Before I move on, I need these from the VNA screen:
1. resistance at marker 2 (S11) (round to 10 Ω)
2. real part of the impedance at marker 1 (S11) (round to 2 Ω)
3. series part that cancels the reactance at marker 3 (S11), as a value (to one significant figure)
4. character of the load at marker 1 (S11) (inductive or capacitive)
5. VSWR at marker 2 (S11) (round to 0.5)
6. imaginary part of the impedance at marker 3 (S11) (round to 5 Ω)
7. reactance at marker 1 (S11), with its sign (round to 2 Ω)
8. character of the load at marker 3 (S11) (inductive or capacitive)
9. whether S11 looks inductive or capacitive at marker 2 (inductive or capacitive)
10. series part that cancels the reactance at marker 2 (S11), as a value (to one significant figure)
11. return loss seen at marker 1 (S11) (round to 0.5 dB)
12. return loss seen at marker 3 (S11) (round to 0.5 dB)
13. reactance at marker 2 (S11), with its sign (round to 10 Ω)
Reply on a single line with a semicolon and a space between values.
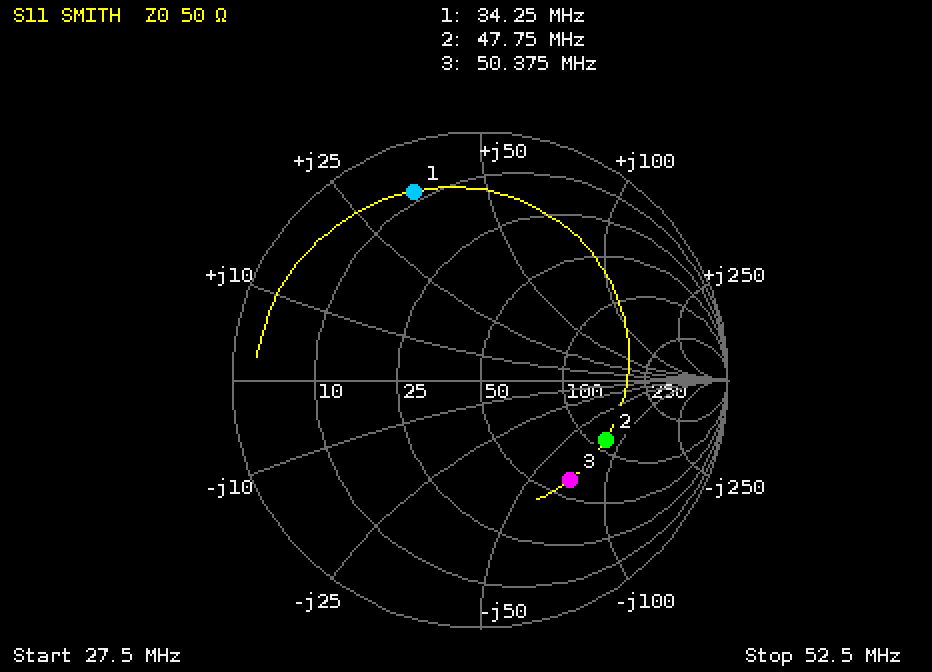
110 Ω; 8 Ω; 200 nH; inductive; 3.5; -70 Ω; +34 Ω; capacitive; capacitive; 300 nH; 2.0 dB; 5.5 dB; -80 Ω
